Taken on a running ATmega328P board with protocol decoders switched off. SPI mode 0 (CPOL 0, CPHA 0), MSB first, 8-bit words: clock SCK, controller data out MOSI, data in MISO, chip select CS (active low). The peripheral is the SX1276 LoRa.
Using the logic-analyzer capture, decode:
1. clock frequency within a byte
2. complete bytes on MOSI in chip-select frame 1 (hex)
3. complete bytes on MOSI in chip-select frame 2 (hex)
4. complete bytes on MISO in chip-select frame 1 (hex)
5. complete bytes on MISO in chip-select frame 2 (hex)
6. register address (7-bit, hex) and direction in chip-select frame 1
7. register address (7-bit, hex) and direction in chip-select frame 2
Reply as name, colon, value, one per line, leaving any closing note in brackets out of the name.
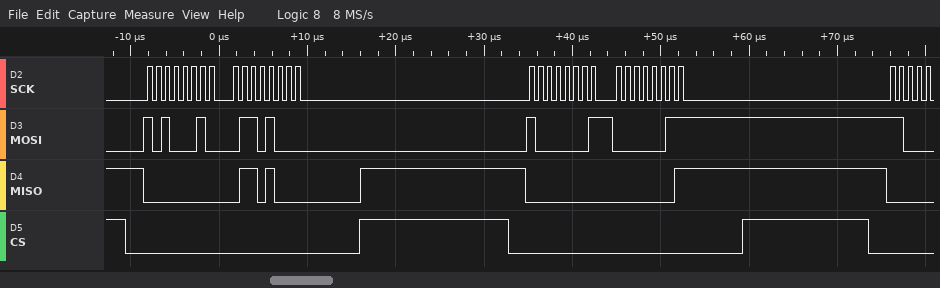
clock frequency within a byte: 1 MHz
complete bytes on MOSI in chip-select frame 1: 0xA2 0x68
complete bytes on MOSI in chip-select frame 2: 0x81 0x03
complete bytes on MISO in chip-select frame 1: 0x00 0x68
complete bytes on MISO in chip-select frame 2: 0x00 0x01
register address (7-bit, hex) and direction in chip-select frame 1: 0x22 write
register address (7-bit, hex) and direction in chip-select frame 2: 0x01 write
